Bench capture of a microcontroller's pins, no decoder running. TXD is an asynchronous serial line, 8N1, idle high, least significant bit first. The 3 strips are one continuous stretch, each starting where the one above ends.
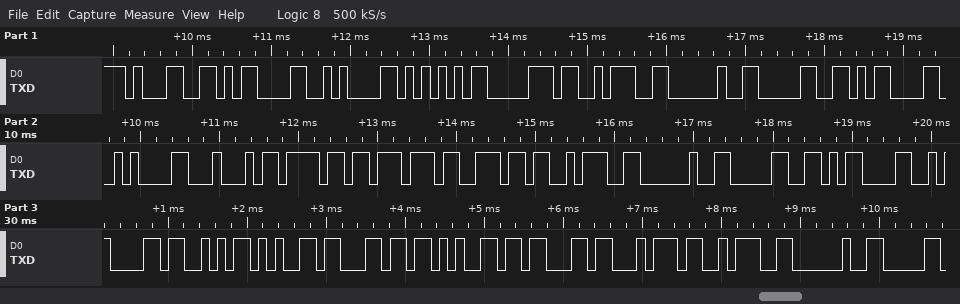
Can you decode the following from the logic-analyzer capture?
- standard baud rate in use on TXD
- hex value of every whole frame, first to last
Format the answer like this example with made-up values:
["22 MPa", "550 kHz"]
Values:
["9600 baud", "31 0D 0A 55 70 3A 20 30 0D 0A 44 6F 77 6E 3A 20 30 0D 0A 53 65 6C 65 63 74 3A 20"]
